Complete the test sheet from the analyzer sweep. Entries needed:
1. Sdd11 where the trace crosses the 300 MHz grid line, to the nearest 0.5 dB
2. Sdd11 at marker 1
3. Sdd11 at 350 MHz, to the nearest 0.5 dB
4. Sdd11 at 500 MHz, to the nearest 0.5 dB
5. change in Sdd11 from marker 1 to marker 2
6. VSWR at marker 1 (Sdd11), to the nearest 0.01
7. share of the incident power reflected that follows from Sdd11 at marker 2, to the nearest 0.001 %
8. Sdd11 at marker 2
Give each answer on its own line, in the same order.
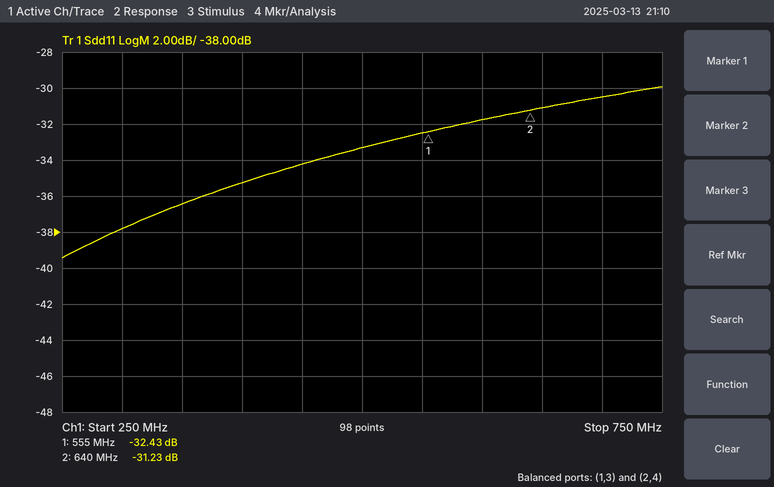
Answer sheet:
-38.0 dB
-32.43 dB
-36.5 dB
-33.5 dB
1.20 dB
1.05
0.075 %
-31.23 dB
